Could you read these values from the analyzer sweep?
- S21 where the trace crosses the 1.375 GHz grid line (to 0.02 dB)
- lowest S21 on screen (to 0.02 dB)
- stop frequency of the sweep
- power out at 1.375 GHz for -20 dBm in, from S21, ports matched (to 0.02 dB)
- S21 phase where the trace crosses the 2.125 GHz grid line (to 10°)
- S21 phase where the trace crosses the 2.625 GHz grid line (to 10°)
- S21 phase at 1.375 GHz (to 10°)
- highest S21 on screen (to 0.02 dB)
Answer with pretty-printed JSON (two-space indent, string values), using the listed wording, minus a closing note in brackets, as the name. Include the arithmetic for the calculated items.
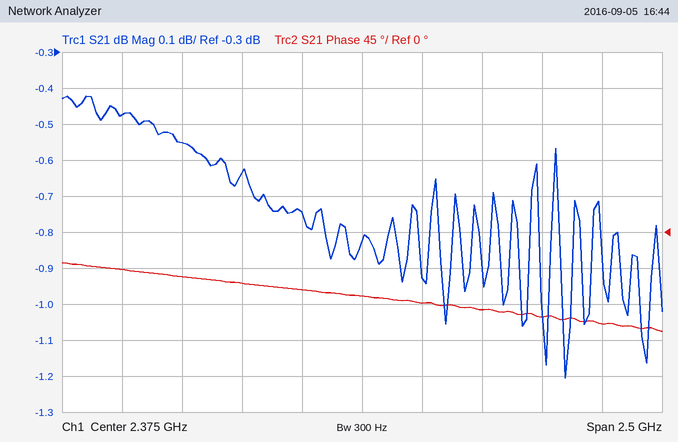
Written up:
{
  "S21 where the trace crosses the 1.375 GHz grid line": "-0.48 dB",
  "lowest S21 on screen": "-1.20 dB",
  "stop frequency of the sweep": "3.625 GHz",
  "power out at 1.375 GHz for -20 dBm in, from S21, ports matched": "-20 dBm + (-0.48 dB) = -20.48 dBm",
  "S21 phase where the trace crosses the 2.125 GHz grid line": "-70°",
  "S21 phase where the trace crosses the 2.625 GHz grid line": "-90°",
  "S21 phase at 1.375 GHz": "-50°",
  "highest S21 on screen": "-0.42 dB"
}
